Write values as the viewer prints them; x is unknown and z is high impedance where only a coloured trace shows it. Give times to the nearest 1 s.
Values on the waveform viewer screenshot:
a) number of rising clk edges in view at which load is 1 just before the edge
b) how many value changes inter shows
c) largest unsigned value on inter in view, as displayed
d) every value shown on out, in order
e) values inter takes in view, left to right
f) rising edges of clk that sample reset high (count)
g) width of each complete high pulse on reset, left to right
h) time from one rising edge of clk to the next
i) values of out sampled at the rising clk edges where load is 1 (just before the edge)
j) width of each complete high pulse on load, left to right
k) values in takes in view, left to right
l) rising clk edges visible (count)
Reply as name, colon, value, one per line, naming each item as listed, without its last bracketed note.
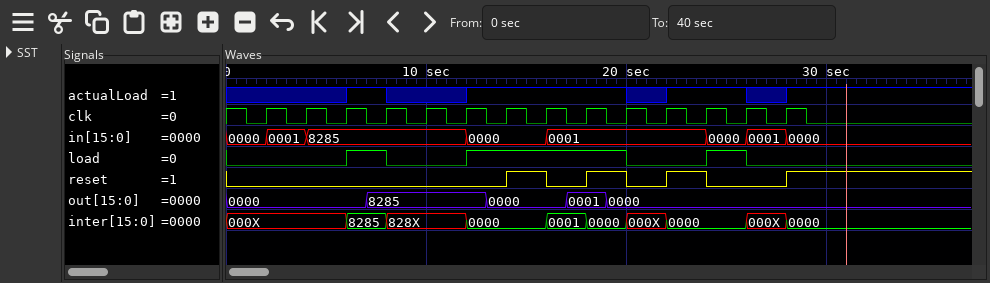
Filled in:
number of rising clk edges in view at which load is 1 just before the edge: 6
how many value changes inter shows: 9
largest unsigned value on inter in view, as displayed: 8285
every value shown on out, in order: 0000, 8285, 0000, 0001, 0000
values inter takes in view, left to right: 000X, 8285, 828X, 0000, 0001, 0000, 000X, 0000, 000X, 0000
rising edges of clk that sample reset high: 3
width of each complete high pulse on reset, left to right: 2 s, 2 s, 2 s
time from one rising edge of clk to the next: 2 s
values of out sampled at the rising clk edges where load is 1: 8285, 0000, 0000, 0001, 0000, 0000
width of each complete high pulse on load, left to right: 2 s, 8 s, 2 s
values in takes in view, left to right: 0000, 0001, 8285, 0000, 0001, 0000, 0001, 0000
rising clk edges visible: 14
